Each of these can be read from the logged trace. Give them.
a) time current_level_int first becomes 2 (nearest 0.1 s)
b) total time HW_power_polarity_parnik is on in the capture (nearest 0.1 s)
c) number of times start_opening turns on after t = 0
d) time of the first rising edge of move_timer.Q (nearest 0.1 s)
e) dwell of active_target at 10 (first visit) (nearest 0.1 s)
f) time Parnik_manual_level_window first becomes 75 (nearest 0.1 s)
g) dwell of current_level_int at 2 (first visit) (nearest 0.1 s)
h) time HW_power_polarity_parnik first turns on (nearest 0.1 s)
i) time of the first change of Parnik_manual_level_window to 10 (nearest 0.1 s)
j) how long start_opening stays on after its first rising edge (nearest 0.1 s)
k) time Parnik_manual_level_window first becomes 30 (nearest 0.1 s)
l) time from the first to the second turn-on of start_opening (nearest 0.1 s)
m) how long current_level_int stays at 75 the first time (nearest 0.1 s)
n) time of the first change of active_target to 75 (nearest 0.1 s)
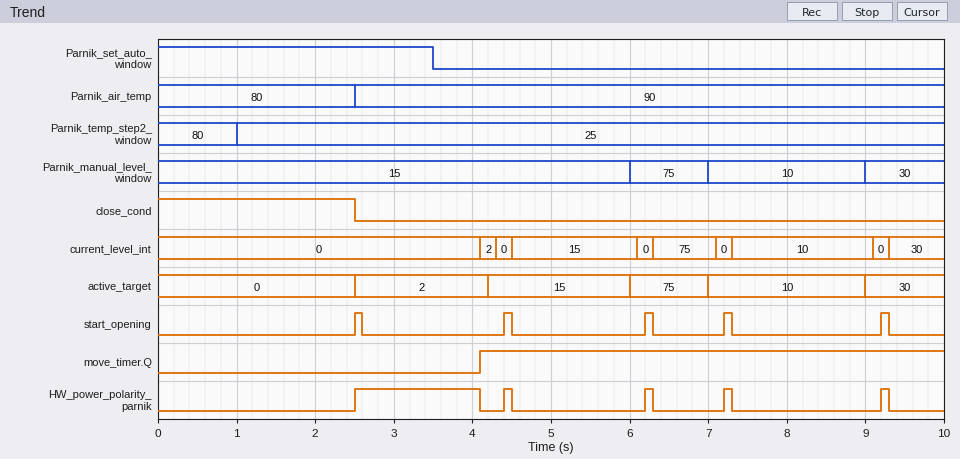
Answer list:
4.1 s
2.0 s
5
4.1 s
2.0 s
6.0 s
0.2 s
2.5 s
7.0 s
0.1 s
9.0 s
1.9 s
0.8 s
6.0 s
